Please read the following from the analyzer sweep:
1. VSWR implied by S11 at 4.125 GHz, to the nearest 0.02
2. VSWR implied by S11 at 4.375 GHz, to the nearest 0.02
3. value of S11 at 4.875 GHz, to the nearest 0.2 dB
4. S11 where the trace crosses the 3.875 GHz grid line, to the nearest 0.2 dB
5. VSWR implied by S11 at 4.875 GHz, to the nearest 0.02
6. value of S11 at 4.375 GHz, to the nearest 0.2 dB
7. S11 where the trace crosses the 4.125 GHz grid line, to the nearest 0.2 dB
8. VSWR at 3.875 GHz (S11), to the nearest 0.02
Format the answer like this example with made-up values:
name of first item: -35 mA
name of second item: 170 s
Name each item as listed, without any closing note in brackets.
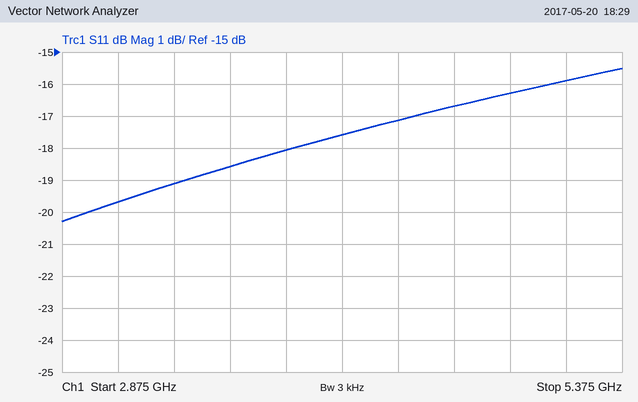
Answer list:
VSWR implied by S11 at 4.125 GHz, to the nearest 0.02: 1.30
VSWR implied by S11 at 4.375 GHz, to the nearest 0.02: 1.32
value of S11 at 4.875 GHz, to the nearest 0.2 dB: -16.2 dB
S11 where the trace crosses the 3.875 GHz grid line, to the nearest 0.2 dB: -18.0 dB
VSWR implied by S11 at 4.875 GHz, to the nearest 0.02: 1.36
value of S11 at 4.375 GHz, to the nearest 0.2 dB: -17.2 dB
S11 where the trace crosses the 4.125 GHz grid line, to the nearest 0.2 dB: -17.6 dB
VSWR at 3.875 GHz (S11), to the nearest 0.02: 1.28
